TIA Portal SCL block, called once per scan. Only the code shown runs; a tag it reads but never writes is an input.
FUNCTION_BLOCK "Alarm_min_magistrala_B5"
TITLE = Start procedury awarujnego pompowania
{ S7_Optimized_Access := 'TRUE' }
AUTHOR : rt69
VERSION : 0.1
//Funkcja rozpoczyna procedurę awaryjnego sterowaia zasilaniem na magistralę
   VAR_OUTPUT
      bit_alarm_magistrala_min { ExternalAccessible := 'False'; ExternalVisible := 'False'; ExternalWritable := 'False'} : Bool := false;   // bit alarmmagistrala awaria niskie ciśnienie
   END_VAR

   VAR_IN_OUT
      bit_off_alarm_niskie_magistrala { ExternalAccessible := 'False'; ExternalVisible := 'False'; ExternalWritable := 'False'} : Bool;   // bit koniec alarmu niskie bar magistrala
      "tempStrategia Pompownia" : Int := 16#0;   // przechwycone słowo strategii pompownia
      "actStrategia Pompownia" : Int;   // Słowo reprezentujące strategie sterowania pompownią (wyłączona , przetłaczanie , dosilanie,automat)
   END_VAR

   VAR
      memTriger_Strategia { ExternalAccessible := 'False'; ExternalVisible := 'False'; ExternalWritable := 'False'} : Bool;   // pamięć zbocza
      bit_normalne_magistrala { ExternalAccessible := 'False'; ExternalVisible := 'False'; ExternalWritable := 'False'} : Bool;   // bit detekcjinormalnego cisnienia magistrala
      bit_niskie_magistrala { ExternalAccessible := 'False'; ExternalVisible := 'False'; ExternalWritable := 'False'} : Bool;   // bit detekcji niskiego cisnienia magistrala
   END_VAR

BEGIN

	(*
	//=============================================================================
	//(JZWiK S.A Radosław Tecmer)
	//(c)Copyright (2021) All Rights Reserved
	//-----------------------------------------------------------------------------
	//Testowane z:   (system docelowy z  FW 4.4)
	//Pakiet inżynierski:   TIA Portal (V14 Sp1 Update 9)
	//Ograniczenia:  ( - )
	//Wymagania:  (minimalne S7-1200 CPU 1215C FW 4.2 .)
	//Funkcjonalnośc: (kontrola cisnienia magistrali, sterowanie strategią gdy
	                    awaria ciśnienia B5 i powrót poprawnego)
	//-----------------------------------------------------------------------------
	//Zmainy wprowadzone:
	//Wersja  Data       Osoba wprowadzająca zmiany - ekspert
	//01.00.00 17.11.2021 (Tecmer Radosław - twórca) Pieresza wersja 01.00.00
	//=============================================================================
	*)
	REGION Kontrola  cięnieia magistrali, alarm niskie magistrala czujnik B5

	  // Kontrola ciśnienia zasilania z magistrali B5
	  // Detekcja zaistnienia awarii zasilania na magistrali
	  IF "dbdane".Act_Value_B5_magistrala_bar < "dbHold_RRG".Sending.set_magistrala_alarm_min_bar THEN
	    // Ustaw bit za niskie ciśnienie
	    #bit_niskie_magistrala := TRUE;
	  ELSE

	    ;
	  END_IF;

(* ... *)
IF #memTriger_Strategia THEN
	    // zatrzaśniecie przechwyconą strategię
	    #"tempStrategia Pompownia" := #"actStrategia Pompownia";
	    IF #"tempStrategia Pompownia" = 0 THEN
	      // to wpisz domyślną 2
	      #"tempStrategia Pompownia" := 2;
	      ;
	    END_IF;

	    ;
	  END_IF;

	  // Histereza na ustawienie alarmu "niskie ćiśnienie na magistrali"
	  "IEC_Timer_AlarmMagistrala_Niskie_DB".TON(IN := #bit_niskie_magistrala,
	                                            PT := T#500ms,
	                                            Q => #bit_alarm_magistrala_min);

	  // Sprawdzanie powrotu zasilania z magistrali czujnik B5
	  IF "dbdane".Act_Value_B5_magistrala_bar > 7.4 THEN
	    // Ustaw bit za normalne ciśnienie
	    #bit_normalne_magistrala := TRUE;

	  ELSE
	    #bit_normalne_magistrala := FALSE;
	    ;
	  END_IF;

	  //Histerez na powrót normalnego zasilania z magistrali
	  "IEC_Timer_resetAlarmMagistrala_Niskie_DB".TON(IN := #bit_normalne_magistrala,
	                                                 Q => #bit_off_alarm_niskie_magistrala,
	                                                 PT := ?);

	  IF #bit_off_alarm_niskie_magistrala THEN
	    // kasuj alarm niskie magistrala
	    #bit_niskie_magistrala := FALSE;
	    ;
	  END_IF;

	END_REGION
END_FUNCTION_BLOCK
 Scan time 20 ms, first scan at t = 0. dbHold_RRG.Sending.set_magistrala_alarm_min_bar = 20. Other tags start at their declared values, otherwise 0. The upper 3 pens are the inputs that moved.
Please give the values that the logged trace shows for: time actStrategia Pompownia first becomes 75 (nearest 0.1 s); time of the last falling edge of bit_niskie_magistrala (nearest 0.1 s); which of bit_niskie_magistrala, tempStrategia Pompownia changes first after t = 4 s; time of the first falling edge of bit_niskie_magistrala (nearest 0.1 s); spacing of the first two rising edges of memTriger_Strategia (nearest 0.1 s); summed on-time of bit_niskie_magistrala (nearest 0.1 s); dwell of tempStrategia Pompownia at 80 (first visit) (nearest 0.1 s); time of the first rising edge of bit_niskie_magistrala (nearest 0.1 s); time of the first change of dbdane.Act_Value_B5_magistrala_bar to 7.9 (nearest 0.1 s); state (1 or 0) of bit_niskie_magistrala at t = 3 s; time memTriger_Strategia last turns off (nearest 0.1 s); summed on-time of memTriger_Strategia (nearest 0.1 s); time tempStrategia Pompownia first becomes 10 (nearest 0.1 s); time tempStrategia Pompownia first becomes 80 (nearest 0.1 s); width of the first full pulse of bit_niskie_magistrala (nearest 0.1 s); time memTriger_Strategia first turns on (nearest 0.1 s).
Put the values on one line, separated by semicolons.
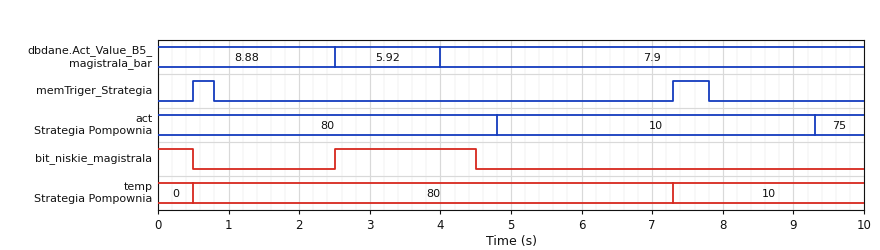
9.3 s; 4.5 s; bit_niskie_magistrala; 0.5 s; 6.8 s; 2.5 s; 6.8 s; 2.5 s; 4.0 s; 1; 7.8 s; 0.8 s; 7.3 s; 0.5 s; 2.0 s; 0.5 s
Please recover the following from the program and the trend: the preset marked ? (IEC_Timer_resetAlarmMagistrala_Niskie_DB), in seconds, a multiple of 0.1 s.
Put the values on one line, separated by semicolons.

0.5 s
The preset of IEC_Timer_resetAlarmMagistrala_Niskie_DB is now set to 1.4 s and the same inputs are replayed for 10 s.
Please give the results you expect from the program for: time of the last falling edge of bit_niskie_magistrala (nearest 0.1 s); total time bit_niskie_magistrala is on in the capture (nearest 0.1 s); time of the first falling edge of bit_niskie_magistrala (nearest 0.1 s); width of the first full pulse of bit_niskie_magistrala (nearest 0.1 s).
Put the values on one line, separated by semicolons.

5.4 s; 4.3 s; 1.4 s; 2.9 s
